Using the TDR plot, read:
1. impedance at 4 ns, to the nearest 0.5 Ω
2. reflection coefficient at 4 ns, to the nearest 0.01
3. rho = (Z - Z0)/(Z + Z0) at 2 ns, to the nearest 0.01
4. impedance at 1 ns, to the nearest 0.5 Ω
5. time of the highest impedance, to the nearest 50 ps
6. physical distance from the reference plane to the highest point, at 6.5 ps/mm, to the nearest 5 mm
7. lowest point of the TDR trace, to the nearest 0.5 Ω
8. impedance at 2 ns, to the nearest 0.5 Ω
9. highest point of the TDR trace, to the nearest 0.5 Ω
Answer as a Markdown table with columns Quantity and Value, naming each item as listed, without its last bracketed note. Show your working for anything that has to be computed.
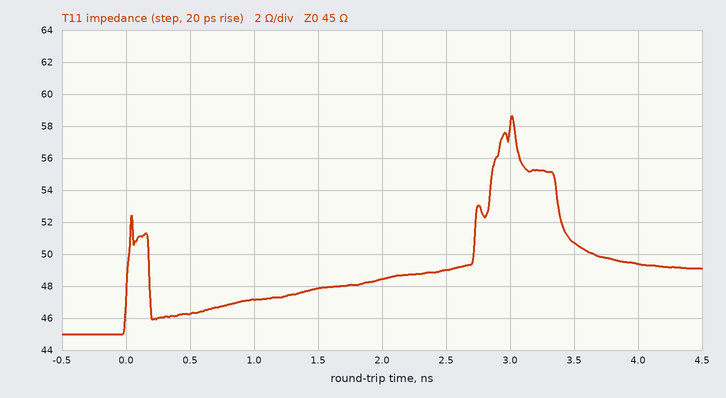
| Quantity | Value |
|---|---|
| impedance at 4 ns, to the nearest 0.5 Ω | 49.5 Ω |
| reflection coefficient at 4 ns, to the nearest 0.01 | (49.5 − 45)/(49.5 + 45) ≈ +0.05 |
| rho = (Z - Z0)/(Z + Z0) at 2 ns, to the nearest 0.01 | (48.5 − 45)/(48.5 + 45) ≈ +0.04 |
| impedance at 1 ns, to the nearest 0.5 Ω | 47.0 Ω |
| time of the highest impedance, to the nearest 50 ps | 3.00 ns |
| physical distance from the reference plane to the highest point, at 6.5 ps/mm, to the nearest 5 mm | 3.00 ns / 2 / 6.5 ps/mm ≈ 231 mm, so 230 mm to the nearest 5 mm |
| lowest point of the TDR trace, to the nearest 0.5 Ω | 45.0 Ω |
| impedance at 2 ns, to the nearest 0.5 Ω | 48.5 Ω |
| highest point of the TDR trace, to the nearest 0.5 Ω | 58.5 Ω |
